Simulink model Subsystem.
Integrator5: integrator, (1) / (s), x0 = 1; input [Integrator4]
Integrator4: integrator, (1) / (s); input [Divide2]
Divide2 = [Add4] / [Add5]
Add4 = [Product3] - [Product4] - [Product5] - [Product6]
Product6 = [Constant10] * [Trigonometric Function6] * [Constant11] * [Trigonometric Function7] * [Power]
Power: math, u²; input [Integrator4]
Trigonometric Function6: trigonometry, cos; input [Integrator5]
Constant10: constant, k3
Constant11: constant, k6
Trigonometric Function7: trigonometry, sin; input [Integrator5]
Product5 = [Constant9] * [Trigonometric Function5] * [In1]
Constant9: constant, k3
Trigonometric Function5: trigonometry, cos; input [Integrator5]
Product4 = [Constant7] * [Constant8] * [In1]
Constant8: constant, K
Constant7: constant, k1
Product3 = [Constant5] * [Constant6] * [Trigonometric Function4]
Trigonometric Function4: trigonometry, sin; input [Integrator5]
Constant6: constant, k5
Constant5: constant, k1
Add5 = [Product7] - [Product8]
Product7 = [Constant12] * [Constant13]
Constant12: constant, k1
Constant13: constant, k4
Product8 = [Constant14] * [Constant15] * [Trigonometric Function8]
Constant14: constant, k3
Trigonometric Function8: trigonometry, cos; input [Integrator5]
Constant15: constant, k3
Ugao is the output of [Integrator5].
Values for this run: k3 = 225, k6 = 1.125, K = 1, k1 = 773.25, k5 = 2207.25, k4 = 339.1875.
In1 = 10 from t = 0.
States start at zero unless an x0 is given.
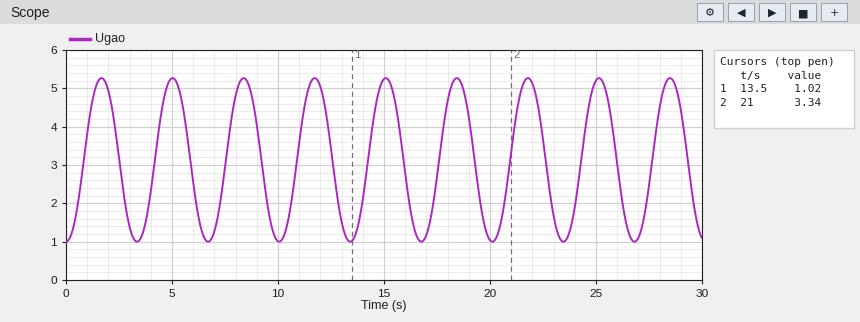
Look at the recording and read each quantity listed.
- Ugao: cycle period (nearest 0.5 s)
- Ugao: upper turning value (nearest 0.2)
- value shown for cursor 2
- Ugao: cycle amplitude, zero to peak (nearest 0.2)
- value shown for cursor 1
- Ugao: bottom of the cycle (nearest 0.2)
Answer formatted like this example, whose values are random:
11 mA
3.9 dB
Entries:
3.5 s
5.2
3.34
2.2
1.02
1.0
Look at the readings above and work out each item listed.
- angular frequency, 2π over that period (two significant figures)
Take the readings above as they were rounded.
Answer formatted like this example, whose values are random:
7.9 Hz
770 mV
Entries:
1.8 rad/s
